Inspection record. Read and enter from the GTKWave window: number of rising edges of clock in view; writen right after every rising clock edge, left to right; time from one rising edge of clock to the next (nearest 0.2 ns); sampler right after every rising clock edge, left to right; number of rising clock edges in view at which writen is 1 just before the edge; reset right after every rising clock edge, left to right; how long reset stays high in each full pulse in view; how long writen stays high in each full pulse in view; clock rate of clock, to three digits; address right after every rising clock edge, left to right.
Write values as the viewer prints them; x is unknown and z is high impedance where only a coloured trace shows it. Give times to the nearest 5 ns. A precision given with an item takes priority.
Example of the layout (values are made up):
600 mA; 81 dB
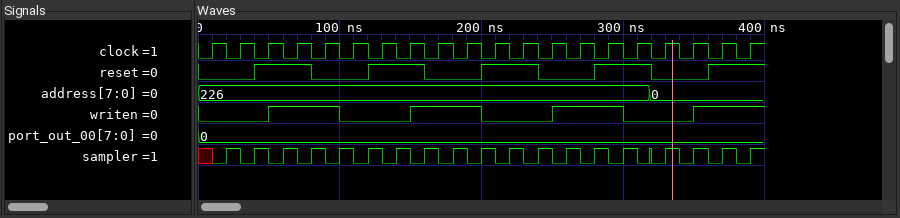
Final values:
20; 0 0 1 1 1 0 0 1 1 1 0 0 1 1 1 0 0 1 1 1; 20 ns; 0 0 0 0 0 0 0 0 0 0 0 0 0 0 0 0 1 1 1 1; 8; 0 0 1 1 0 0 1 1 0 0 1 1 0 0 1 1 0 0 1 1; 40 ns, 40 ns, 40 ns, 40 ns; 50 ns, 50 ns, 50 ns; 50.0 MHz; 226, 226, 226, 226, 226, 226, 226, 226, 226, 226, 226, 226, 226, 226, 226, 226, 0, 0, 0, 0
